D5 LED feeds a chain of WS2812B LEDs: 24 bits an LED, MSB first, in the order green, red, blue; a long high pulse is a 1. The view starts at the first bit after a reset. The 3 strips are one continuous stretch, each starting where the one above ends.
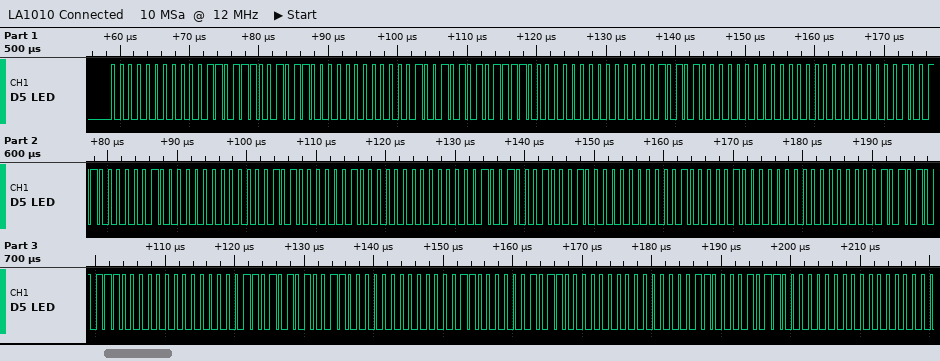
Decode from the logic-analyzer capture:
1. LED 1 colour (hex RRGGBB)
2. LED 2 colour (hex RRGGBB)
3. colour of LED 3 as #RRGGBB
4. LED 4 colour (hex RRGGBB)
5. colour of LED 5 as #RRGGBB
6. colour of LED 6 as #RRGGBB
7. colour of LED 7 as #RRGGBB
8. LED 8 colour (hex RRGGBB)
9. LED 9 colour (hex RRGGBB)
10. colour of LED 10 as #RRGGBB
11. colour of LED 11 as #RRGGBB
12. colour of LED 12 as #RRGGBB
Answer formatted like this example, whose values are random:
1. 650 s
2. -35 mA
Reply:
1. #1B0096
2. #1200AF
3. #010050
4. #000013
5. #00020A
6. #000409
7. #001110
8. #00402A
9. #007035
10. #004C18
11. #001603
12. #000B00
